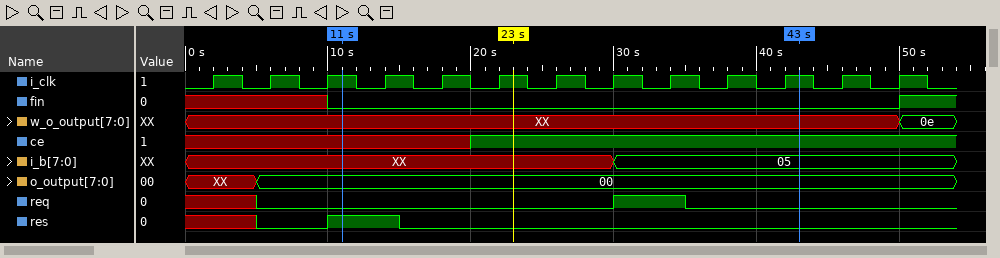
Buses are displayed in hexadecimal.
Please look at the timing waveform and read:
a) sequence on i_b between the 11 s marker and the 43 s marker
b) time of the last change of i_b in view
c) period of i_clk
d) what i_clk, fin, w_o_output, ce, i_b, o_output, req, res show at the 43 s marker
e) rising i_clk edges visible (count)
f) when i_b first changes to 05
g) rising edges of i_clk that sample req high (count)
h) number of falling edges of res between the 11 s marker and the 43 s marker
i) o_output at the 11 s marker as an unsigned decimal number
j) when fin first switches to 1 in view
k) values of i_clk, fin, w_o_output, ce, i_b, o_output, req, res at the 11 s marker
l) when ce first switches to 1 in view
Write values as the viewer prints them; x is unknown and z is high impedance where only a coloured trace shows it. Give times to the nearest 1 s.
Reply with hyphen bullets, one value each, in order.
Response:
- XX, 05
- 30 s
- 4 s
- i_clk=1, fin=0, w_o_output=XX, ce=1, i_b=05, o_output=00, req=0, res=0
- 13
- 30 s
- 1
- 1
- 0
- 50 s
- i_clk=1, fin=0, w_o_output=XX, ce=x, i_b=XX, o_output=00, req=0, res=1
- 20 s
